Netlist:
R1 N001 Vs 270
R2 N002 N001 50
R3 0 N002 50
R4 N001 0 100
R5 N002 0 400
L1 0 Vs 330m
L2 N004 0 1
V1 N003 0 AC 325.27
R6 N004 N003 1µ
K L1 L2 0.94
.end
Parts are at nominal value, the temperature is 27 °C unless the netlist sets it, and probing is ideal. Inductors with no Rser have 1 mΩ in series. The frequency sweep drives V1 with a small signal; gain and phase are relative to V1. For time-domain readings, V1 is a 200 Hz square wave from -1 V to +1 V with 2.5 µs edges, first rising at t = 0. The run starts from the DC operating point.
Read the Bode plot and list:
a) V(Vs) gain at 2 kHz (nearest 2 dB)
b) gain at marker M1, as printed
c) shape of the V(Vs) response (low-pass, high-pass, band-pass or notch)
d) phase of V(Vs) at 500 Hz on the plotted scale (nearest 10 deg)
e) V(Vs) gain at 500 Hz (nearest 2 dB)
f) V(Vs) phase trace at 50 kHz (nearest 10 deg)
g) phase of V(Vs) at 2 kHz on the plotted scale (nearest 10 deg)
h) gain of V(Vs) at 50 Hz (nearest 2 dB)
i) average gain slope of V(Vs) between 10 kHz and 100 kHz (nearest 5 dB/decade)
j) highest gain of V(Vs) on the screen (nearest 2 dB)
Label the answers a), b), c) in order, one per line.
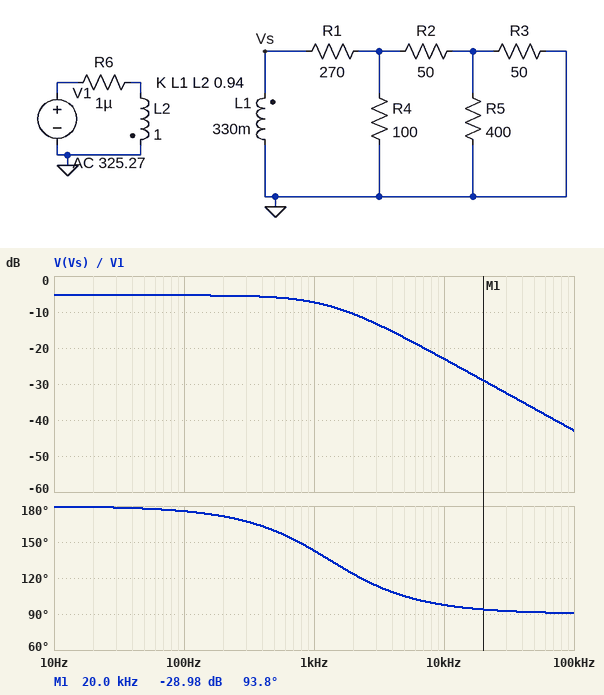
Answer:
a) -10 dB
b) -28.98 dB
c) low-pass
d) 160 deg
e) -6 dB
f) 90 deg
g) 120 deg
h) -6 dB
i) -20 dB/decade
j) -6 dB
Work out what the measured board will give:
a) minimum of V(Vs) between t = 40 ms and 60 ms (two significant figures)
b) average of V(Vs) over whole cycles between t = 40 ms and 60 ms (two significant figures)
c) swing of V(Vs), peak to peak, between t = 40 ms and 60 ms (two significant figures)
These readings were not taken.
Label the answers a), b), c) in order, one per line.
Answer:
a) -1.1 V
b) -540 mV
c) 1.1 V
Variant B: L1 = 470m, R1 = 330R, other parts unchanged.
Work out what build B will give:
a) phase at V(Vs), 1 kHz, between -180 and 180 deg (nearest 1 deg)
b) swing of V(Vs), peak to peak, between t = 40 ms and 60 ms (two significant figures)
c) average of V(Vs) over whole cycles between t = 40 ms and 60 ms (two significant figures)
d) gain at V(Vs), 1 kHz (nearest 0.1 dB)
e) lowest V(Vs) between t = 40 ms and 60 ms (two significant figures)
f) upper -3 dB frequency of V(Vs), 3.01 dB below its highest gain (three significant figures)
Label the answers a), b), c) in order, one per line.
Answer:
a) 138 deg
b) 1.3 V
c) -640 mV
d) -6.4 dB
e) -1.3 V
f) 1.10 kHz
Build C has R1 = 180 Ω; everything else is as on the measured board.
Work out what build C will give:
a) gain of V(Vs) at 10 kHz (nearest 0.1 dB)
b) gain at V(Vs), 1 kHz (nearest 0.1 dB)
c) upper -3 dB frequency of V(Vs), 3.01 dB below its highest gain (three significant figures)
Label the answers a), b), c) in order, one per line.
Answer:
a) -25.9 dB
b) -8.6 dB
c) 947 Hz
